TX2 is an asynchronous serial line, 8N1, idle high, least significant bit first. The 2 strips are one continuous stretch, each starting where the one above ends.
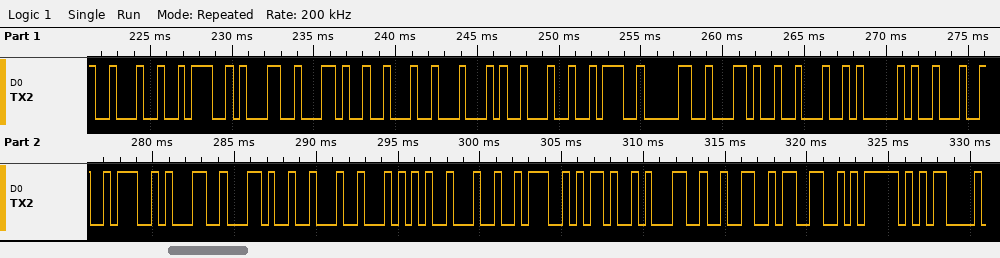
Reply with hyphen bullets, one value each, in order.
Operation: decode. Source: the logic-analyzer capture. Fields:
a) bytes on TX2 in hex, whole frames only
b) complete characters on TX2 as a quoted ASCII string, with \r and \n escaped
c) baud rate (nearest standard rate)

- 22 3A 31 2C 22 44 22 3A 30 2C 22 41 22 3A 31 2C 22 54 22 3A 2D 31 32 33 7D 0D
- "\":1,\"D\":0,\"A\":1,\"T\":-123}\r"
- 2400 baud
